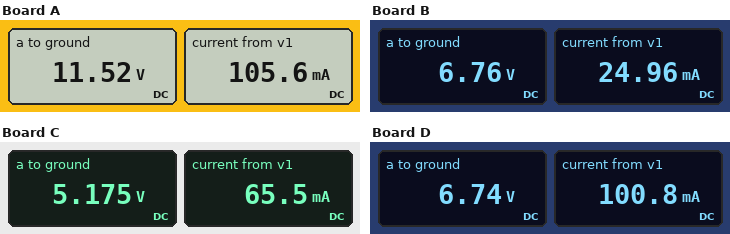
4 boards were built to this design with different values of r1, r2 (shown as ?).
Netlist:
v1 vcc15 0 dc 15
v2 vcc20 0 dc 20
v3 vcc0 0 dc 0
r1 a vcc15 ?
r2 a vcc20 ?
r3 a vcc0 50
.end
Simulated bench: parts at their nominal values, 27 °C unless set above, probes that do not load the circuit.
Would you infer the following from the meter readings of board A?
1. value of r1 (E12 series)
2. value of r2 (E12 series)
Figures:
33 Ω
68 Ω
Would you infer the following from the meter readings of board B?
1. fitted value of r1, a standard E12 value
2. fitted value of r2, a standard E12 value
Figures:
330 Ω
120 Ω
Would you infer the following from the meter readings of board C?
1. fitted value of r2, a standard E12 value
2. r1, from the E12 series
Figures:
390 Ω
150 Ω
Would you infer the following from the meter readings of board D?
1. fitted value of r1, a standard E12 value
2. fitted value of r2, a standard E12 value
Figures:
82 Ω
390 Ω
